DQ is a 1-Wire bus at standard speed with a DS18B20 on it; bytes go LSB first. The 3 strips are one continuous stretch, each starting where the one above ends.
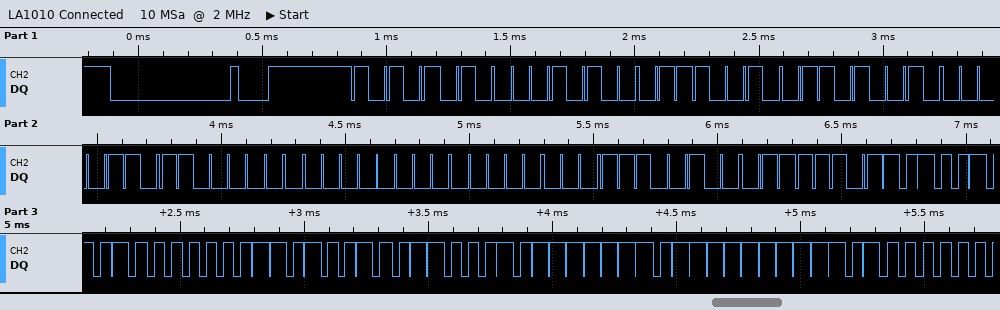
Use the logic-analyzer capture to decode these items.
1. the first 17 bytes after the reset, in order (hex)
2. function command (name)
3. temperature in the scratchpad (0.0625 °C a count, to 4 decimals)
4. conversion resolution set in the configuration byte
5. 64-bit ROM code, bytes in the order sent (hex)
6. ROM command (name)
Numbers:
55 28 4E 96 60 03 00 00 27 BE 25 01 4B 46 7F FF 0B
Read Scratchpad
18.3125 °C
12 bits
28 4E 96 60 03 00 00 27
Match ROM
